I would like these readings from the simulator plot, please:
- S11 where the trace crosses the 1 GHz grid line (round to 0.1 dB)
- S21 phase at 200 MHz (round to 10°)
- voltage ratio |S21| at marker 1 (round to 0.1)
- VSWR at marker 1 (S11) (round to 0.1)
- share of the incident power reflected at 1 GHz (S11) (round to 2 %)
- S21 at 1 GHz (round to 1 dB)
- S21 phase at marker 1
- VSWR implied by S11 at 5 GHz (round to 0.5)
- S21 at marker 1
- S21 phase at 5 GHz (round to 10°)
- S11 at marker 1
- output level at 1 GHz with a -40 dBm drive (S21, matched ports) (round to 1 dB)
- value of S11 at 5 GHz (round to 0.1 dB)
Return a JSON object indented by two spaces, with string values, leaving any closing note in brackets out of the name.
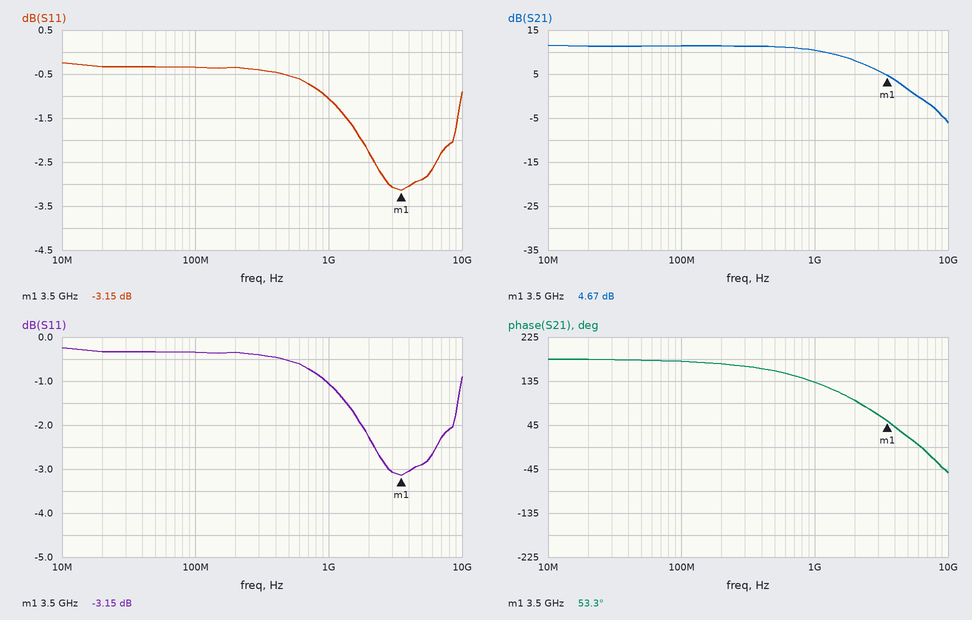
{
  "S11 where the trace crosses the 1 GHz grid line": "-1.1 dB",
  "S21 phase at 200 MHz": "170°",
  "voltage ratio |S21| at marker 1": "1.7",
  "VSWR at marker 1 (S11)": "5.6",
  "share of the incident power reflected at 1 GHz (S11)": "78 %",
  "S21 at 1 GHz": "10 dB",
  "S21 phase at marker 1": "53.3°",
  "VSWR implied by S11 at 5 GHz": "6.0",
  "S21 at marker 1": "4.67 dB",
  "S21 phase at 5 GHz": "20°",
  "S11 at marker 1": "-3.15 dB",
  "output level at 1 GHz with a -40 dBm drive (S21, matched ports)": "-30 dBm",
  "value of S11 at 5 GHz": "-2.9 dB"
}
